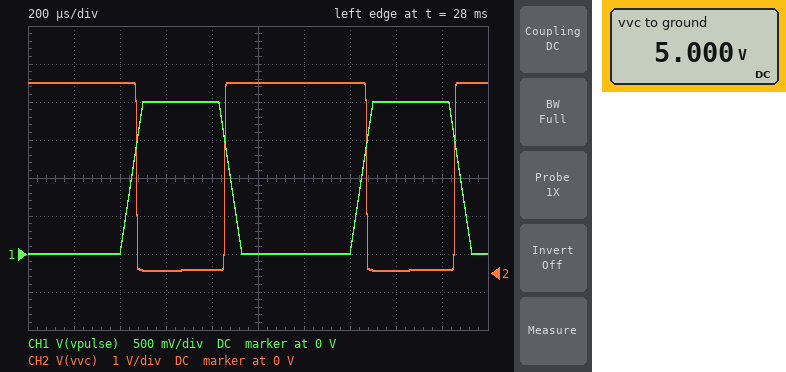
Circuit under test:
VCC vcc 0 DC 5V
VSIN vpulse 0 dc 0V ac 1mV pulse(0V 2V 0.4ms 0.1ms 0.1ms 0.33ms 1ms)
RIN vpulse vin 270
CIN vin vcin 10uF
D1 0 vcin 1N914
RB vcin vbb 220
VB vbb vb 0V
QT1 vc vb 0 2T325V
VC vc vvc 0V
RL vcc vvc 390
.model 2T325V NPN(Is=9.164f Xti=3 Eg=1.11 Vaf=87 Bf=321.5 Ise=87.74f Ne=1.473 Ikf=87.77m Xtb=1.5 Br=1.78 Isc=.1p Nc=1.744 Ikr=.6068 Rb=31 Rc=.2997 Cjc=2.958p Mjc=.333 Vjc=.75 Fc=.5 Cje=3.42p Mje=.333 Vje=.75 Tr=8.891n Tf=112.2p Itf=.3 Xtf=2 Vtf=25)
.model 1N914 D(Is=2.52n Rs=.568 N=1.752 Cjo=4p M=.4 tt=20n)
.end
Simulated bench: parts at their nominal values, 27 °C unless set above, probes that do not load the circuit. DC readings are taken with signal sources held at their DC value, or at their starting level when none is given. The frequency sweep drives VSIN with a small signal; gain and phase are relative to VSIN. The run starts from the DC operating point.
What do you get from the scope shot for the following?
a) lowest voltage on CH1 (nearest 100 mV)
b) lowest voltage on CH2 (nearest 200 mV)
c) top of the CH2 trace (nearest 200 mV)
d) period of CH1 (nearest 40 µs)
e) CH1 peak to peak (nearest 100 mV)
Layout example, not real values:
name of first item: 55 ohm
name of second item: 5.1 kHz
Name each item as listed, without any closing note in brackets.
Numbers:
lowest voltage on CH1: 0 V
lowest voltage on CH2: 0 V
top of the CH2 trace: 5.0 V
period of CH1: 1.00 ms
CH1 peak to peak: 2.0 V
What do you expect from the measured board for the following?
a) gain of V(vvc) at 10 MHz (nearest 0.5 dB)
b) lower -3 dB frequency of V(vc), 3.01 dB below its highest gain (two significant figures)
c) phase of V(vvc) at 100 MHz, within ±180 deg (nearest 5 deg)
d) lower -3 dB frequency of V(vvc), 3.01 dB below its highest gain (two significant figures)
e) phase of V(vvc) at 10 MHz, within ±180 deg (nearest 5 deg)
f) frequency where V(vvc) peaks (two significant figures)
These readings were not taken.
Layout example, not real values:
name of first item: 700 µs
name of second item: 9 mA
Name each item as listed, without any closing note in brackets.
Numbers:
gain of V(vvc) at 10 MHz: -29.0 dB
lower -3 dB frequency of V(vc), 3.01 dB below its highest gain: 35 MHz
phase of V(vvc) at 100 MHz, within ±180 deg: -5 deg
lower -3 dB frequency of V(vvc), 3.01 dB below its highest gain: 35 MHz
phase of V(vvc) at 10 MHz, within ±180 deg: 75 deg
frequency where V(vvc) peaks: 110 MHz
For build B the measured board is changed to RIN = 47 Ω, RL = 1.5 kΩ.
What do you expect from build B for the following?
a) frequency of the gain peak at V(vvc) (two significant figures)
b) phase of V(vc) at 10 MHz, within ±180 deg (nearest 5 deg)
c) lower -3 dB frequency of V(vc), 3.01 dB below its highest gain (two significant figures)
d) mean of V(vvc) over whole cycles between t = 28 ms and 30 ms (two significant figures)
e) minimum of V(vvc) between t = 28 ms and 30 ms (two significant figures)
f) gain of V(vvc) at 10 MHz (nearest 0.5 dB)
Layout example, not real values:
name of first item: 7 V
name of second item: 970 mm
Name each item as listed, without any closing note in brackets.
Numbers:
frequency of the gain peak at V(vvc): 100 MHz
phase of V(vc) at 10 MHz, within ±180 deg: 75 deg
lower -3 dB frequency of V(vc), 3.01 dB below its highest gain: 37 MHz
mean of V(vvc) over whole cycles between t = 28 ms and 30 ms: 3.0 V
minimum of V(vvc) between t = 28 ms and 30 ms: 26 mV
gain of V(vvc) at 10 MHz: -17.0 dB
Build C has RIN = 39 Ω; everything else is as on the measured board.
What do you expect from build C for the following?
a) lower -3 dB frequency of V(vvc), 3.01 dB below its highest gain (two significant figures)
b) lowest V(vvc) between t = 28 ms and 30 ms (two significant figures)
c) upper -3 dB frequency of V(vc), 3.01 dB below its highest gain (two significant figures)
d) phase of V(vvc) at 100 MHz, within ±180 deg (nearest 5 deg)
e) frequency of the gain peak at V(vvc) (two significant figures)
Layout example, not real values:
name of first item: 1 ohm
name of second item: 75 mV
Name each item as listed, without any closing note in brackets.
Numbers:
lower -3 dB frequency of V(vvc), 3.01 dB below its highest gain: 68 MHz
lowest V(vvc) between t = 28 ms and 30 ms: 50 mV
upper -3 dB frequency of V(vc), 3.01 dB below its highest gain: 540 MHz
phase of V(vvc) at 100 MHz, within ±180 deg: 25 deg
frequency of the gain peak at V(vvc): 200 MHz
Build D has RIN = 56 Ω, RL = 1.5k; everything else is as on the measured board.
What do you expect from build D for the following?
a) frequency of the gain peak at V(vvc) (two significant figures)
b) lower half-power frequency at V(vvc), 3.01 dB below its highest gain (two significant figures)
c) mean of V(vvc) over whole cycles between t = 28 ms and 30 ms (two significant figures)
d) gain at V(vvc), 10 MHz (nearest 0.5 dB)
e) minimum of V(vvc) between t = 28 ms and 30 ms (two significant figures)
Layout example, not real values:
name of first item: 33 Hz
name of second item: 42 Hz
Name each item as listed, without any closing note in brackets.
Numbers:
frequency of the gain peak at V(vvc): 99 MHz
lower half-power frequency at V(vvc), 3.01 dB below its highest gain: 36 MHz
mean of V(vvc) over whole cycles between t = 28 ms and 30 ms: 3.0 V
gain at V(vvc), 10 MHz: -17.0 dB
minimum of V(vvc) between t = 28 ms and 30 ms: 26 mV
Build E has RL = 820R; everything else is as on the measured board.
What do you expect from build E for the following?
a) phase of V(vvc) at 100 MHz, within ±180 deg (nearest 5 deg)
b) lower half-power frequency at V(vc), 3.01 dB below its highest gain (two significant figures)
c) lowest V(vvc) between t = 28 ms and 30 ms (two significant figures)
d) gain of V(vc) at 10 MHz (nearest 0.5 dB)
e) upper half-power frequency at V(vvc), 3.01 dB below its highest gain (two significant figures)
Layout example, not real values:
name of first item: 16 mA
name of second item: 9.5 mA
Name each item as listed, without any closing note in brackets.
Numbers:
phase of V(vvc) at 100 MHz, within ±180 deg: -20 deg
lower half-power frequency at V(vc), 3.01 dB below its highest gain: 30 MHz
lowest V(vvc) between t = 28 ms and 30 ms: 46 mV
gain of V(vc) at 10 MHz: -22.5 dB
upper half-power frequency at V(vvc), 3.01 dB below its highest gain: 220 MHz
